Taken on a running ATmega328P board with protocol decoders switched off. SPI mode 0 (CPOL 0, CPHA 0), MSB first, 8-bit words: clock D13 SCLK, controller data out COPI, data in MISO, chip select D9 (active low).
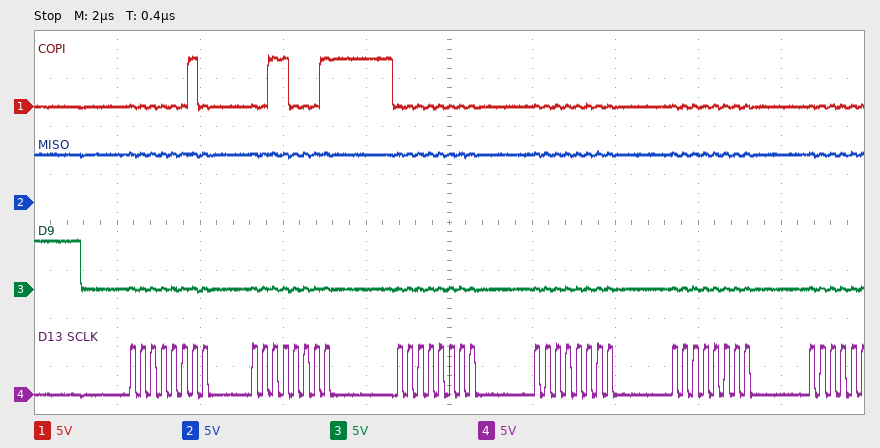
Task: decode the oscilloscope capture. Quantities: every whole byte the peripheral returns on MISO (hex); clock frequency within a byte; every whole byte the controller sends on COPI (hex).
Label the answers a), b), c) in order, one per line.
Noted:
a) FF FF FF FF FF
b) 4 MHz
c) 02 31 00 00 00
